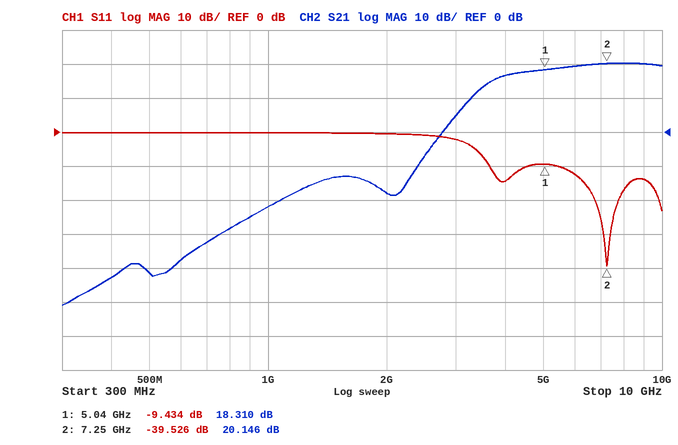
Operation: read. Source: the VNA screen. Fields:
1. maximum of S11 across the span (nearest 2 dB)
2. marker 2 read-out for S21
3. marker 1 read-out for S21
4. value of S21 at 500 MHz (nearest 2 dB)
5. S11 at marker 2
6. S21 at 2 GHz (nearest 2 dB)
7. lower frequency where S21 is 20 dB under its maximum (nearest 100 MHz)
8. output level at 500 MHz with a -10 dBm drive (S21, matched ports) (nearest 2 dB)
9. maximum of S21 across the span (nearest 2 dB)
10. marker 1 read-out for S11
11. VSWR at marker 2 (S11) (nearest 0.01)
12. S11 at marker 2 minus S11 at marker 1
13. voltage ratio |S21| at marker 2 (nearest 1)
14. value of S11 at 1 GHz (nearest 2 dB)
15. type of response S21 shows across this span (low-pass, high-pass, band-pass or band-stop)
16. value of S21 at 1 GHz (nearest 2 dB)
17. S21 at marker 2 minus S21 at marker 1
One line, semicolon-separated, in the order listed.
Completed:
0 dB; 20.146 dB; 18.310 dB; -42 dB; -39.526 dB; -18 dB; 2.8 GHz; -52 dBm; 20 dB; -9.434 dB; 1.02; -30.092 dB; 10; 0 dB; high-pass; -22 dB; 1.836 dB
